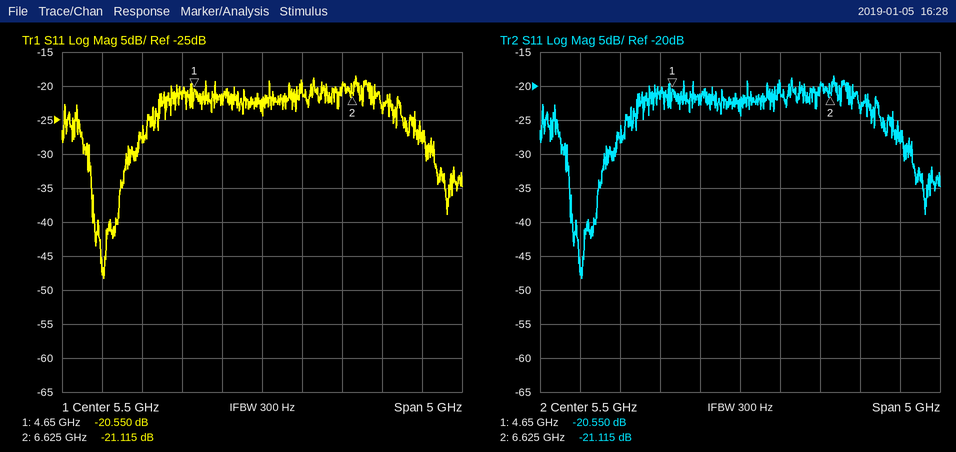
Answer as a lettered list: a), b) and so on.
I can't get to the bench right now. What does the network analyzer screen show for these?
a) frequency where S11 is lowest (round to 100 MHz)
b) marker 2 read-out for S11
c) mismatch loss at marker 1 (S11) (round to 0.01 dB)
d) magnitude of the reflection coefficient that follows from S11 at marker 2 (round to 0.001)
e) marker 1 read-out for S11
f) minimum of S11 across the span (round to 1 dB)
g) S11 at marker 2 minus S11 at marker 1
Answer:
a) 3.5 GHz
b) -21.115 dB
c) 0.04 dB
d) 0.088
e) -20.550 dB
f) -48 dB
g) -0.565 dB
